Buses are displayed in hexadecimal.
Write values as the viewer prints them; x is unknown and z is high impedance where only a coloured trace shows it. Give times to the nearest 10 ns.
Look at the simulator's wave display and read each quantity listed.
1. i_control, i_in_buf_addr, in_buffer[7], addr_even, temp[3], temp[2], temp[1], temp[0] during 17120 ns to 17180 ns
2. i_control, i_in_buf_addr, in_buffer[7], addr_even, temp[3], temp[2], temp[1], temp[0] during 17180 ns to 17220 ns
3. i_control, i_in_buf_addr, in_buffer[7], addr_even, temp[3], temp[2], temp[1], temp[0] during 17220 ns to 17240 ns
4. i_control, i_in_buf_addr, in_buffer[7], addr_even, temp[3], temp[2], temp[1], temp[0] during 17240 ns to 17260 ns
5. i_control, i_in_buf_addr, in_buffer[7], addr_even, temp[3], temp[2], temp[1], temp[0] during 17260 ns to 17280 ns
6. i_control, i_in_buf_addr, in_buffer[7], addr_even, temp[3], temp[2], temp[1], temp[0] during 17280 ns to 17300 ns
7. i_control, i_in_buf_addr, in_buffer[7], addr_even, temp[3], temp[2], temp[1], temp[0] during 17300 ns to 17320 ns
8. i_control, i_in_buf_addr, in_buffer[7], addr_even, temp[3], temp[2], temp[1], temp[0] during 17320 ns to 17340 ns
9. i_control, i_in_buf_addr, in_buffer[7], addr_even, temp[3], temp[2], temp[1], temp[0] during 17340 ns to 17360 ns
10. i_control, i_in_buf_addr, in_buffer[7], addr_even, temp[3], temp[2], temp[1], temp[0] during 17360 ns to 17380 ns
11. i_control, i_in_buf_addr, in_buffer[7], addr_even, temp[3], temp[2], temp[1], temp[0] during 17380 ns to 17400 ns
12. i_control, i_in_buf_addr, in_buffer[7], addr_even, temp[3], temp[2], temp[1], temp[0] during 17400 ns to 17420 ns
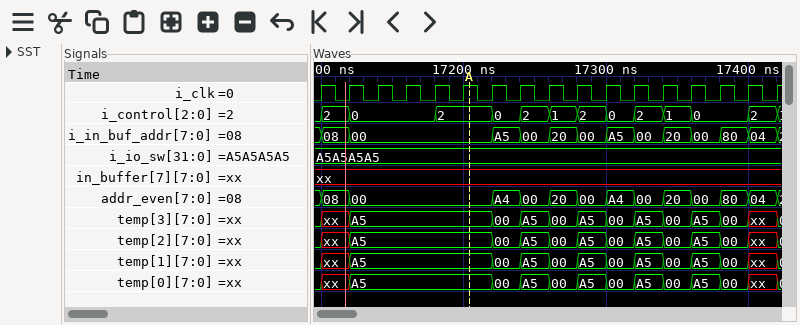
i_control=0, i_in_buf_addr=00, in_buffer[7]=xx, addr_even=00, temp[3]=A5, temp[2]=A5, temp[1]=A5, temp[0]=A5
i_control=2, i_in_buf_addr=00, in_buffer[7]=xx, addr_even=00, temp[3]=A5, temp[2]=A5, temp[1]=A5, temp[0]=A5
i_control=0, i_in_buf_addr=A5, in_buffer[7]=xx, addr_even=A4, temp[3]=00, temp[2]=00, temp[1]=00, temp[0]=00
i_control=2, i_in_buf_addr=00, in_buffer[7]=xx, addr_even=00, temp[3]=A5, temp[2]=A5, temp[1]=A5, temp[0]=A5
i_control=1, i_in_buf_addr=20, in_buffer[7]=xx, addr_even=20, temp[3]=00, temp[2]=00, temp[1]=00, temp[0]=00
i_control=2, i_in_buf_addr=00, in_buffer[7]=xx, addr_even=00, temp[3]=A5, temp[2]=A5, temp[1]=A5, temp[0]=A5
i_control=0, i_in_buf_addr=A5, in_buffer[7]=xx, addr_even=A4, temp[3]=00, temp[2]=00, temp[1]=00, temp[0]=00
i_control=2, i_in_buf_addr=00, in_buffer[7]=xx, addr_even=00, temp[3]=A5, temp[2]=A5, temp[1]=A5, temp[0]=A5
i_control=1, i_in_buf_addr=20, in_buffer[7]=xx, addr_even=20, temp[3]=00, temp[2]=00, temp[1]=00, temp[0]=00
i_control=0, i_in_buf_addr=00, in_buffer[7]=xx, addr_even=00, temp[3]=A5, temp[2]=A5, temp[1]=A5, temp[0]=A5
i_control=0, i_in_buf_addr=80, in_buffer[7]=xx, addr_even=80, temp[3]=00, temp[2]=00, temp[1]=00, temp[0]=00
i_control=2, i_in_buf_addr=04, in_buffer[7]=xx, addr_even=04, temp[3]=xx, temp[2]=xx, temp[1]=xx, temp[0]=xx
